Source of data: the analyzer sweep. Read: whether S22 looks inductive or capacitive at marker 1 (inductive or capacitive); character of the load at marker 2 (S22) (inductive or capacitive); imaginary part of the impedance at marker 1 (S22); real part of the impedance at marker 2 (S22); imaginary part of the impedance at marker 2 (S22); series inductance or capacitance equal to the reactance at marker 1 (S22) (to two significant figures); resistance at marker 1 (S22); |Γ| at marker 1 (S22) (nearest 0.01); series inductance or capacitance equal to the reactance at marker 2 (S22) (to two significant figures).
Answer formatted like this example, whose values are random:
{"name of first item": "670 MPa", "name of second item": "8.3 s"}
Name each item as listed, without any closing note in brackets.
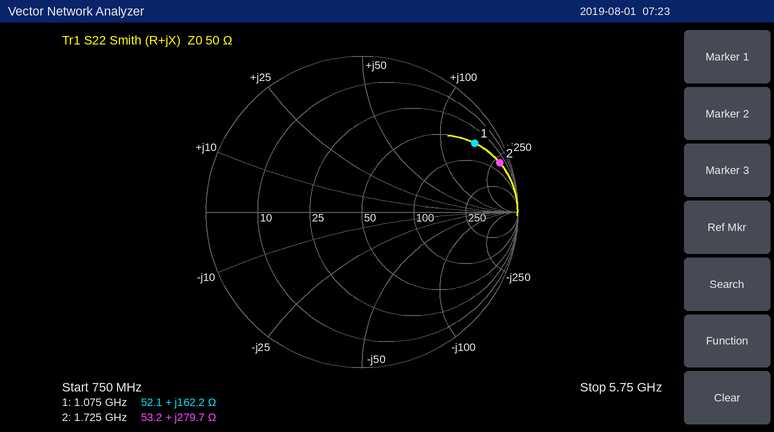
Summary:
{"whether S22 looks inductive or capacitive at marker 1": "inductive", "character of the load at marker 2 (S22)": "inductive", "imaginary part of the impedance at marker 1": "+162.2 Ω", "real part of the impedance at marker 2": "53.2 Ω", "imaginary part of the impedance at marker 2": "+279.7 Ω", "series inductance or capacitance equal to the reactance at marker 1 (S22)": "24 nH", "resistance at marker 1": "52.1 Ω", "|Γ| at marker 1 (S22)": "0.85", "series inductance or capacitance equal to the reactance at marker 2 (S22)": "26 nH"}
